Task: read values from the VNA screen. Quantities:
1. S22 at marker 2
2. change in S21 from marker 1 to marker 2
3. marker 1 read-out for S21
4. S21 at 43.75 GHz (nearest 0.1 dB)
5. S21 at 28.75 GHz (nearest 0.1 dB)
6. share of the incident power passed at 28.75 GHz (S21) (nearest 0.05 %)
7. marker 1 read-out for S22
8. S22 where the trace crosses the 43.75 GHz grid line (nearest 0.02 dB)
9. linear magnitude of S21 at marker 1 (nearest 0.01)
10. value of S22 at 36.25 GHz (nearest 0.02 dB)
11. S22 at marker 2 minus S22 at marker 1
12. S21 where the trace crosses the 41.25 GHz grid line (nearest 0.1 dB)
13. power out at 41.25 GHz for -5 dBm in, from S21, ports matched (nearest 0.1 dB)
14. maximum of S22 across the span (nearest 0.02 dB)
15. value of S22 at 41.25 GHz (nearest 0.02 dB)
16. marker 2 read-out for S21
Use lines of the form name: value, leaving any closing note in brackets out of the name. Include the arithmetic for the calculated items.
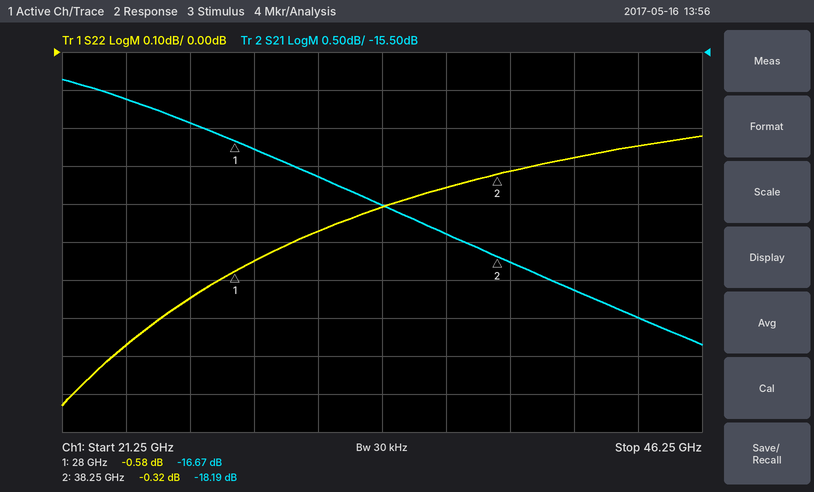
S22 at marker 2: -0.32 dB
change in S21 from marker 1 to marker 2: -18.19 − (-16.67) = -1.52 dB
marker 1 read-out for S21: -16.67 dB
S21 at 43.75 GHz: -19.0 dB
S21 at 28.75 GHz: -16.8 dB
share of the incident power passed at 28.75 GHz (S21): 10^(-16.8/10) ≈ 2.09 %, so 2.10 % to the nearest 0.05 %
marker 1 read-out for S22: -0.58 dB
S22 where the trace crosses the 43.75 GHz grid line: -0.24 dB
linear magnitude of S21 at marker 1: 10^(-16.67/20) ≈ 0.15
value of S22 at 36.25 GHz: -0.36 dB
S22 at marker 2 minus S22 at marker 1: -0.32 − (-0.58) = 0.26 dB
S21 where the trace crosses the 41.25 GHz grid line: -18.6 dB
power out at 41.25 GHz for -5 dBm in, from S21, ports matched: -5 dBm + (-18.6 dB) = -23.6 dBm
maximum of S22 across the span: -0.22 dB
value of S22 at 41.25 GHz: -0.28 dB
marker 2 read-out for S21: -18.19 dB
